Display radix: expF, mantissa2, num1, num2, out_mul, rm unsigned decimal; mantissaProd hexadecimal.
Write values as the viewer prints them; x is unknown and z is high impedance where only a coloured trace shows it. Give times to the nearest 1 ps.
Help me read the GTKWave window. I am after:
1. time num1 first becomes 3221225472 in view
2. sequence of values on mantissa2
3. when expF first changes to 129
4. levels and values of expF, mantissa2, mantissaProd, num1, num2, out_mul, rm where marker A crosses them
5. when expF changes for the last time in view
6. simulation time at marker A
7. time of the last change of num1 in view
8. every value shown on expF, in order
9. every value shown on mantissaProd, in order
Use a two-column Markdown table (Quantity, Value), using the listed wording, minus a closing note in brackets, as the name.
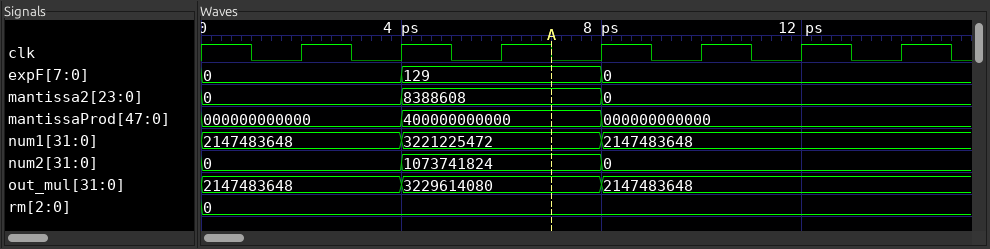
| Quantity | Value |
|---|---|
| time num1 first becomes 3221225472 in view | 4 ps |
| sequence of values on mantissa2 | 0, 8388608, 0 |
| when expF first changes to 129 | 4 ps |
| levels and values of expF, mantissa2, mantissaProd, num1, num2, out_mul, rm where marker A crosses them | expF=129, mantissa2=8388608, mantissaProd=400000000000, num1=3221225472, num2=1073741824, out_mul=3229614080, rm=0 |
| when expF changes for the last time in view | 8 ps |
| simulation time at marker A | 7 ps |
| time of the last change of num1 in view | 8 ps |
| every value shown on expF, in order | 0, 129, 0 |
| every value shown on mantissaProd, in order | 000000000000, 400000000000, 000000000000 |
